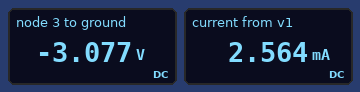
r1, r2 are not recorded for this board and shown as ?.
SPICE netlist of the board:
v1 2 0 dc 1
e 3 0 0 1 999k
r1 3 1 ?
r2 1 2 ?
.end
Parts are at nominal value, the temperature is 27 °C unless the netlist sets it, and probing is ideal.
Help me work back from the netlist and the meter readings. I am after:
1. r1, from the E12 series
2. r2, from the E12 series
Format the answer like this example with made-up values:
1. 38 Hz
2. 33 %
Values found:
1. 1.2 kΩ
2. 390 Ω
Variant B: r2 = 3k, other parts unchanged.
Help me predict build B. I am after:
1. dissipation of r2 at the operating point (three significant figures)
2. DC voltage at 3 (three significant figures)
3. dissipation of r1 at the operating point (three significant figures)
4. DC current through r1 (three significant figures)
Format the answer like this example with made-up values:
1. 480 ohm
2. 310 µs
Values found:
1. 333 µW
2. -400 mV
3. 133 µW
4. 333 µA
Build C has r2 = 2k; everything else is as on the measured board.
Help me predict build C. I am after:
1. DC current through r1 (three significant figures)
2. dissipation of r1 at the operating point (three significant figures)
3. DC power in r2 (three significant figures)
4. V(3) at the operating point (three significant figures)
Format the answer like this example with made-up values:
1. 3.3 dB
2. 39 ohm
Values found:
1. 500 µA
2. 300 µW
3. 500 µW
4. -600 mV
